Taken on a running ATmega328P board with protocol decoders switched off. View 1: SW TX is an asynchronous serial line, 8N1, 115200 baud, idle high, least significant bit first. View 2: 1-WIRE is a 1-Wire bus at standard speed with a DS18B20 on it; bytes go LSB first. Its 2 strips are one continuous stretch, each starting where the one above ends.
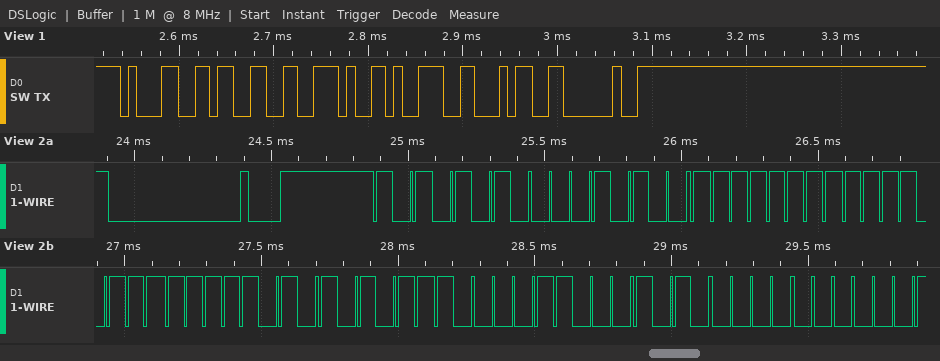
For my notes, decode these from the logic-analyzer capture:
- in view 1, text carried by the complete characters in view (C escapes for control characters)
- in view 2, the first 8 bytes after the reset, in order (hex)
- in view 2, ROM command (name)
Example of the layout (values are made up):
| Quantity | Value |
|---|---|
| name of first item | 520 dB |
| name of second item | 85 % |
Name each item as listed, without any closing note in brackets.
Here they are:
| Quantity | Value |
|---|---|
| in view 1, text carried by the complete characters in view | "13.94 " |
| in view 2, the first 8 bytes after the reset, in order | 55 28 FF EF 5F 75 18 05 |
| in view 2, ROM command | Match ROM |
